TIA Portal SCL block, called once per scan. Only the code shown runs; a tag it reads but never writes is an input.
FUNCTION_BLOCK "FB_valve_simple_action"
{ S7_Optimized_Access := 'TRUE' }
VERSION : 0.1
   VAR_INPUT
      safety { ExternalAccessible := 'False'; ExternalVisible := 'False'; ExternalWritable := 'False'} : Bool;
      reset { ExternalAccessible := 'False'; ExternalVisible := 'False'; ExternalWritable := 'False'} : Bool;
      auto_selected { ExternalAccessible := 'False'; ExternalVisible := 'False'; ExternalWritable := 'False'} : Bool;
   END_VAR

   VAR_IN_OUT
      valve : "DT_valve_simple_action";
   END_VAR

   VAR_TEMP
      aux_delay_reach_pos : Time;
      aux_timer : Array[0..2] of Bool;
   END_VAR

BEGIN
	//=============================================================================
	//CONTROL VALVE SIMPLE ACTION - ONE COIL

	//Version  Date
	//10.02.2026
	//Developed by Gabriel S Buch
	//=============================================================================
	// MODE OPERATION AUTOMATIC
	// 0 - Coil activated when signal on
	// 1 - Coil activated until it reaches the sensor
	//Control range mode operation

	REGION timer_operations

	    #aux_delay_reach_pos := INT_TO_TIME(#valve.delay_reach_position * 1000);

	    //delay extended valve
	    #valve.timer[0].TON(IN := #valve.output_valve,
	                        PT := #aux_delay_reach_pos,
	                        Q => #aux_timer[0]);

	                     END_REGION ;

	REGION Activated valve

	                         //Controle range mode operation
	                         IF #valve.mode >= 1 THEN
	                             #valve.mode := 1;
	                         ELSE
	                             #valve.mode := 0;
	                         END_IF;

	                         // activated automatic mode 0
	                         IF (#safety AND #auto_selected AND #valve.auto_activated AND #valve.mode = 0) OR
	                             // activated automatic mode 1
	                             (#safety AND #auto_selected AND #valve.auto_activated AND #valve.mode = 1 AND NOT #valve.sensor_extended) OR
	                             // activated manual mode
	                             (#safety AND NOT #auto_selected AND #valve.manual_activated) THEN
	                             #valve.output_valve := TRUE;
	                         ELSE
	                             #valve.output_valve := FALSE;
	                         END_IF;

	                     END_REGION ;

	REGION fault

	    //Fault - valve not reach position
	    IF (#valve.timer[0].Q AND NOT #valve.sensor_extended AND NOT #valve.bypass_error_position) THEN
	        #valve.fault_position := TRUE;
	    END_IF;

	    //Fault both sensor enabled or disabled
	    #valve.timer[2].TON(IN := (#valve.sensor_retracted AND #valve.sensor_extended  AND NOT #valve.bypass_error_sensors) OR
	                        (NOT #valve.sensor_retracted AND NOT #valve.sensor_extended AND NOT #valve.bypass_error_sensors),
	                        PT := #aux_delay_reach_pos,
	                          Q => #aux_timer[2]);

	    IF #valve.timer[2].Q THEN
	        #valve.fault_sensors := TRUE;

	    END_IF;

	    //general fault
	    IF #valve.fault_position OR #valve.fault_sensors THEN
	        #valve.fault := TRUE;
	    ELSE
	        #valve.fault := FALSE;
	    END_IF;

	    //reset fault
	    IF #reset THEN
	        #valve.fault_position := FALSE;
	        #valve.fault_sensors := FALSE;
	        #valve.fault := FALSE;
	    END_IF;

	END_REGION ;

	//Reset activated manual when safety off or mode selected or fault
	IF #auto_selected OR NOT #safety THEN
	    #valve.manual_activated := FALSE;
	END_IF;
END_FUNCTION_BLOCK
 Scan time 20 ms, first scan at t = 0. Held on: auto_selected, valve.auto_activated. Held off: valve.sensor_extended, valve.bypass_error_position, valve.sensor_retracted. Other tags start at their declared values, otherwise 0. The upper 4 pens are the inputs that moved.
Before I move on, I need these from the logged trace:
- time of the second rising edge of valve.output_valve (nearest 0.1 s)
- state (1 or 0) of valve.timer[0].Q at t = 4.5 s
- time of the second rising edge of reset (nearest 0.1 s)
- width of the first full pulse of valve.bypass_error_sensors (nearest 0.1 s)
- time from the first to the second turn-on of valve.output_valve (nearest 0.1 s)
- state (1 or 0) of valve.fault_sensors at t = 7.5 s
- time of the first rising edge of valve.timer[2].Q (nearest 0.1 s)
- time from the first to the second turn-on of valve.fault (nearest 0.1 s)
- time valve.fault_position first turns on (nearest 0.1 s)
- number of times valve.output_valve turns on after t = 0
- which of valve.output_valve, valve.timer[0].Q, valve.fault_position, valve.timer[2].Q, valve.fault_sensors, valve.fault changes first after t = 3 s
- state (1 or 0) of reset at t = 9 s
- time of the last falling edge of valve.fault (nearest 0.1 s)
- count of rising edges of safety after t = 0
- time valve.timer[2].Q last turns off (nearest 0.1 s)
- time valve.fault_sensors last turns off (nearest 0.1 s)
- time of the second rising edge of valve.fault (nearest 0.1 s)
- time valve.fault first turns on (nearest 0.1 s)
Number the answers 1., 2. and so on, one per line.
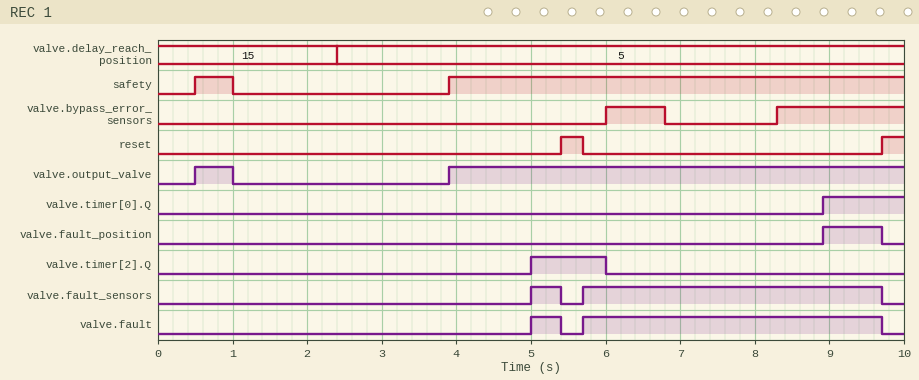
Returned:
1. 3.9 s
2. 0
3. 9.7 s
4. 0.8 s
5. 3.4 s
6. 1
7. 5.0 s
8. 0.7 s
9. 8.9 s
10. 2
11. valve.output_valve
12. 0
13. 9.7 s
14. 2
15. 6.0 s
16. 9.7 s
17. 5.7 s
18. 5.0 s
